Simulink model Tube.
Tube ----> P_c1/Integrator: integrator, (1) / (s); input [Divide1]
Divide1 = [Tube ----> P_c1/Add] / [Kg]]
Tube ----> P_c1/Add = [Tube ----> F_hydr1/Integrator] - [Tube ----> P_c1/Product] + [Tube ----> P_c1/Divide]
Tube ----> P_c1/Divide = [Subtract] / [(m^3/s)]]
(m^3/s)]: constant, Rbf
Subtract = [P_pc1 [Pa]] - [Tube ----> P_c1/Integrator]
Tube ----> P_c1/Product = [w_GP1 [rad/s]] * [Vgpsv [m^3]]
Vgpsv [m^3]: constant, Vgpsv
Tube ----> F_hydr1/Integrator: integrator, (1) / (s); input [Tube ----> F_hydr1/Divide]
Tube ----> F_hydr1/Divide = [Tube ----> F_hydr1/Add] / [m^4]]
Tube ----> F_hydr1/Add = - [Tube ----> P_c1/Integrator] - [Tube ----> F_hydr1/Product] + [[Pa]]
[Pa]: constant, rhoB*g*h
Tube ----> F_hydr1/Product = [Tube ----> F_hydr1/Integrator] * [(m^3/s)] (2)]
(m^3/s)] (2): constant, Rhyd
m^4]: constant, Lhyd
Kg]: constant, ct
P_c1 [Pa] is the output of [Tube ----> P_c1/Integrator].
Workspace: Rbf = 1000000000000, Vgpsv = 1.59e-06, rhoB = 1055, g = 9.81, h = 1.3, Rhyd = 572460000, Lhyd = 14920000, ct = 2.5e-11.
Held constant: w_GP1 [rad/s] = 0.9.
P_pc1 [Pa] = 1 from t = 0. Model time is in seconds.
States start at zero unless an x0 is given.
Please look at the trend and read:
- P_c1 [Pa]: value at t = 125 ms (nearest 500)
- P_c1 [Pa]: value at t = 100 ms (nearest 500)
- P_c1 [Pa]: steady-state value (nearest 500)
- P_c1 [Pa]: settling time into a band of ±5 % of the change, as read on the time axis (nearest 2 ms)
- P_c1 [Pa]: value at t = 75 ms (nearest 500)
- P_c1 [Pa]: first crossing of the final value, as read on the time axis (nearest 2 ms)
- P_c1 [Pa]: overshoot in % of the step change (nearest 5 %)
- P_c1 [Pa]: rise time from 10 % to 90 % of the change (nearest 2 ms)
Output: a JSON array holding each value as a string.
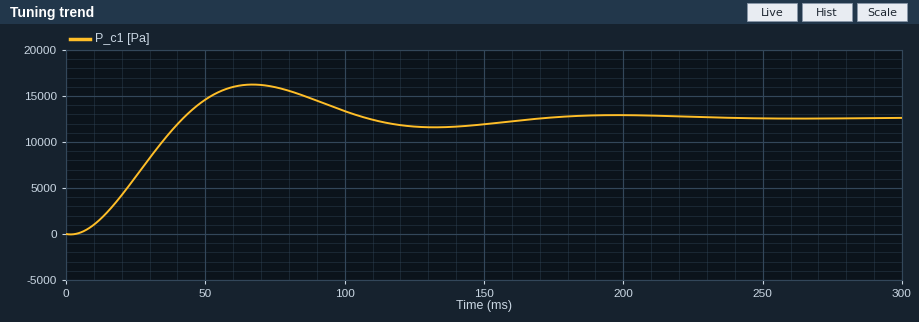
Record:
["11500", "13500", "12500", "152 ms", "16000", "42 ms", "30 %", "28 ms"]
